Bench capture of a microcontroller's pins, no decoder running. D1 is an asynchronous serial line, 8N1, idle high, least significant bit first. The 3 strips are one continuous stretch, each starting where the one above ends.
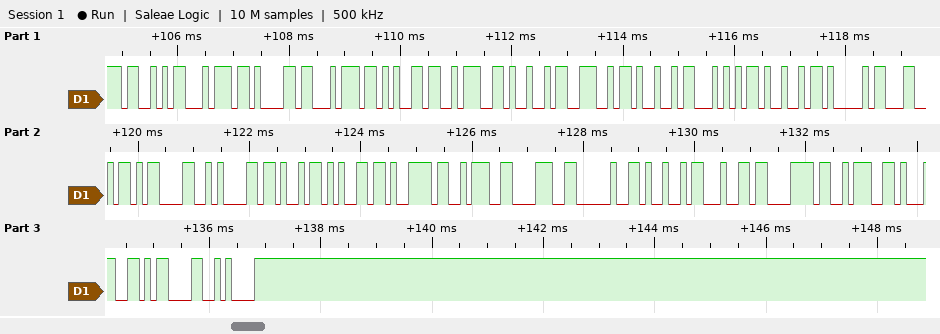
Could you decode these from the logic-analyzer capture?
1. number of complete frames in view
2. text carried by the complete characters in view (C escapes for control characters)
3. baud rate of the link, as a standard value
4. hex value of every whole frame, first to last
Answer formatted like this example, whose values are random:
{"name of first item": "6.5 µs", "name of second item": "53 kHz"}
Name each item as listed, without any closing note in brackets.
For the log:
{"number of complete frames in view": "28", "text carried by the complete characters in view": "\"State:INITIAL\\r\\nKey:8 Idx:1\\r\\n\"", "baud rate of the link, as a standard value": "9600 baud", "hex value of every whole frame, first to last": "53 74 61 74 65 3A 49 4E 49 54 49 41 4C 0D 0A 4B 65 79 3A 38 20 49 64 78 3A 31 0D 0A"}
